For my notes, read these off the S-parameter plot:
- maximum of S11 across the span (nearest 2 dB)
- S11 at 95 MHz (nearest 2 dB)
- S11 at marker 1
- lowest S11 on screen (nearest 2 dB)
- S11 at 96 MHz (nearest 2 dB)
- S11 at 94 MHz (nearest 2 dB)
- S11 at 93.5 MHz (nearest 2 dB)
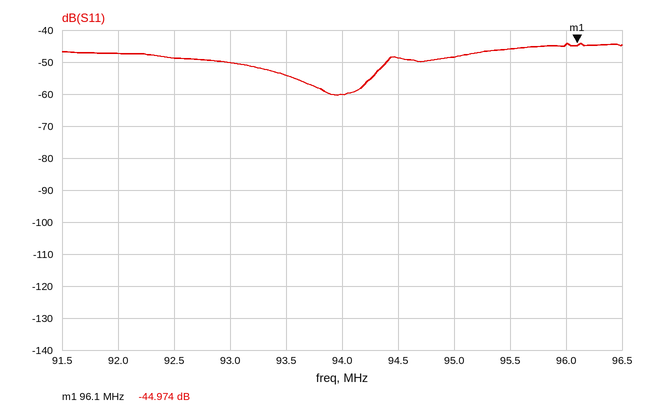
-44 dB
-48 dB
-44.974 dB
-60 dB
-44 dB
-60 dB
-54 dB
